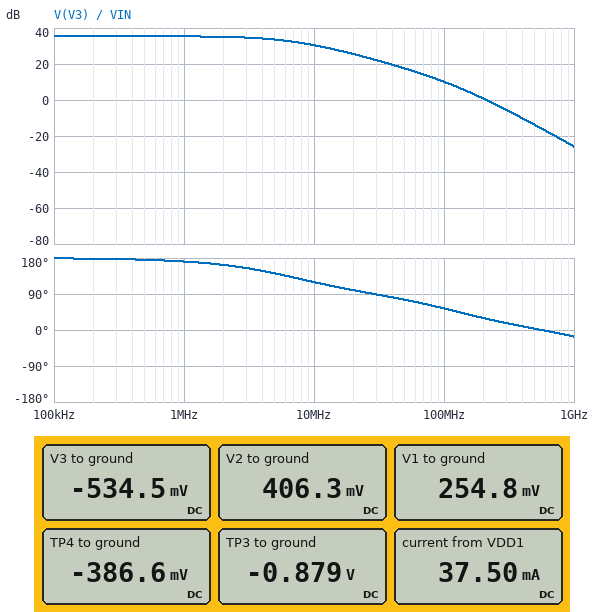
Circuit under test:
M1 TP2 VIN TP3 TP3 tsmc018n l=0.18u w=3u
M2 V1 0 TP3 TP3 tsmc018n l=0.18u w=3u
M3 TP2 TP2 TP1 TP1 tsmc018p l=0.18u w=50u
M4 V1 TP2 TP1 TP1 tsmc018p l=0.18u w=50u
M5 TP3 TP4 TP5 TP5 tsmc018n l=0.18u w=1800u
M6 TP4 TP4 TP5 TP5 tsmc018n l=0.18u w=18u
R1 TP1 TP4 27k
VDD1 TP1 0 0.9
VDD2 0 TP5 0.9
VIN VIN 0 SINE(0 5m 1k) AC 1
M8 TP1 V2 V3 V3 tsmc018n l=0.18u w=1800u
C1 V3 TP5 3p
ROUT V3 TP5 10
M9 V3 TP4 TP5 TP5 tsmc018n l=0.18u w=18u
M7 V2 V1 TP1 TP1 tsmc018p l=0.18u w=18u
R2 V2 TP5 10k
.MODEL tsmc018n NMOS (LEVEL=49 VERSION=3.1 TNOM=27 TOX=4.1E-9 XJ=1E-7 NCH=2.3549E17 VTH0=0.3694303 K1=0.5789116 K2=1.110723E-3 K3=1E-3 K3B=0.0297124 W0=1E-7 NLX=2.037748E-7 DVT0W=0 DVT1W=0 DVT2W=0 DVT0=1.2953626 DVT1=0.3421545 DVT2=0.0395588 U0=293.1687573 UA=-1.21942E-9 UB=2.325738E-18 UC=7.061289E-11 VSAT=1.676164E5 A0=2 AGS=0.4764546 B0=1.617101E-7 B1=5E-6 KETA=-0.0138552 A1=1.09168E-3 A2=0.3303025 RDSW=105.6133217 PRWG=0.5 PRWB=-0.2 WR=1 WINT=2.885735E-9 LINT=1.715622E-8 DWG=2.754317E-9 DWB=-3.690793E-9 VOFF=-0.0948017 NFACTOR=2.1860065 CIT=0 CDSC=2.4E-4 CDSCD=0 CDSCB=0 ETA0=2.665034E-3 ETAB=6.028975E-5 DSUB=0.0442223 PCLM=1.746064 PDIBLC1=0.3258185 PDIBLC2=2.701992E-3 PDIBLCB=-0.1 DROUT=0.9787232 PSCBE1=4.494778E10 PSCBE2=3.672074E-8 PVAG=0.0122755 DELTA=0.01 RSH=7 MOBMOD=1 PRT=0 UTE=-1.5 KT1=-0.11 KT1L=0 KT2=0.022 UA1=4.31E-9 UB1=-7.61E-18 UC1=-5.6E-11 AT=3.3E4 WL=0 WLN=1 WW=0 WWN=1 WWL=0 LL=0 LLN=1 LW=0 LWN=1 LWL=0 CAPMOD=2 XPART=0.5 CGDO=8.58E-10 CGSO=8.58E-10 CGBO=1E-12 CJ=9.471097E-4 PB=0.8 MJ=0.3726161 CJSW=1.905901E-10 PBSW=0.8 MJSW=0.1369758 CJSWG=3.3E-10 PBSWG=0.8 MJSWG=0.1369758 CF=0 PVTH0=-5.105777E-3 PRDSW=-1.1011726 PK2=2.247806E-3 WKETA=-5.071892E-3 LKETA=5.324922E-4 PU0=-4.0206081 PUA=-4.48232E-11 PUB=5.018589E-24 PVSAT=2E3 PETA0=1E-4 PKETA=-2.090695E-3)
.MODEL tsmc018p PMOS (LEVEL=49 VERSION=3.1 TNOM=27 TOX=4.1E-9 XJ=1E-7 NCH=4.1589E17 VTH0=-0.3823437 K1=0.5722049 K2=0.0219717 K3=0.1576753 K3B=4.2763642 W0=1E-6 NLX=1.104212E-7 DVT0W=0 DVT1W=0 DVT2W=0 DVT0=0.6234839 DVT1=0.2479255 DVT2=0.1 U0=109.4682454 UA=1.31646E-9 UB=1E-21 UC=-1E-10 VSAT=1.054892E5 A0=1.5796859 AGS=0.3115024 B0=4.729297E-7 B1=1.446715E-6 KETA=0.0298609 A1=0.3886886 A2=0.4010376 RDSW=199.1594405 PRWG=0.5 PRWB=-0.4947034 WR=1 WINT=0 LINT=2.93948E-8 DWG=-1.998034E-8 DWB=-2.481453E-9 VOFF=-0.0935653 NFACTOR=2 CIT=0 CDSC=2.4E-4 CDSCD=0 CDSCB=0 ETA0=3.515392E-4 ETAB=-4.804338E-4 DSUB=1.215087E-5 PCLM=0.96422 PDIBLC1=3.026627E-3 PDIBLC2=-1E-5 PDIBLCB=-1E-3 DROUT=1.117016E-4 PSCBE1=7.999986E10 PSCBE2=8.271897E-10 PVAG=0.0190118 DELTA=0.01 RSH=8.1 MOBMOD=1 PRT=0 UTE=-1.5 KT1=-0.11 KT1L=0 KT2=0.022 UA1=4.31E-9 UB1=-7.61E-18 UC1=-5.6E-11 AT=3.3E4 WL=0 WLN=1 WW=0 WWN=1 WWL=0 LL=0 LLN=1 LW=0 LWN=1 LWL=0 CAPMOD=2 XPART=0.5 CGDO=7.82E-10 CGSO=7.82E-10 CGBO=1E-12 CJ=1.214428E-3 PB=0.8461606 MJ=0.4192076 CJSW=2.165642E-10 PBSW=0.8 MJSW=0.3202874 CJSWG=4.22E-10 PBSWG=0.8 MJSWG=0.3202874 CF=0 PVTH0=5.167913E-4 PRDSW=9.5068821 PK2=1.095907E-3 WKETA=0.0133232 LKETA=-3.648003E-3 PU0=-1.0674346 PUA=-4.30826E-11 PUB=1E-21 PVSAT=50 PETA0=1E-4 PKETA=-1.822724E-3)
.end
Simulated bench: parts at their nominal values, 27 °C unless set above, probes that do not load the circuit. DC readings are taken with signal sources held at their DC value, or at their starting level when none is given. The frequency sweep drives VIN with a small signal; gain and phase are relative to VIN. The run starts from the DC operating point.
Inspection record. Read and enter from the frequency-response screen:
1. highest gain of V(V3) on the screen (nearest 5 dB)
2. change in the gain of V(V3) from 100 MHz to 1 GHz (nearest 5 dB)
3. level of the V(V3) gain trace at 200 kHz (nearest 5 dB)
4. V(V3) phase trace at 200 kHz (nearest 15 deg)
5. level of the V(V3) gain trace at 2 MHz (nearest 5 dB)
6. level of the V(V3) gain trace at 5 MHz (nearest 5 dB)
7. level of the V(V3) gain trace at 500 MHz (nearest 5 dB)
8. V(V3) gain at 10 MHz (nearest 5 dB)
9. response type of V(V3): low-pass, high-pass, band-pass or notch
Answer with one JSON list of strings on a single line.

["35 dB", "-35 dB", "35 dB", "180 deg", "35 dB", "35 dB", "-15 dB", "30 dB", "low-pass"]
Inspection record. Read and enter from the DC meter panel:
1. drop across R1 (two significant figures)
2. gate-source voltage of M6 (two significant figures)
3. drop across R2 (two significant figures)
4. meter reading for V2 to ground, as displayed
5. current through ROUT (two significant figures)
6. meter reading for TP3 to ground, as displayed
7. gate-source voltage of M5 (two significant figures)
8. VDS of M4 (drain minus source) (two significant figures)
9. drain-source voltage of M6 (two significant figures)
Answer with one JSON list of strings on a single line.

["1.3 V", "510 mV", "1.3 V", "406.3 mV", "37 mA", "-0.879 V", "510 mV", "-650 mV", "510 mV"]
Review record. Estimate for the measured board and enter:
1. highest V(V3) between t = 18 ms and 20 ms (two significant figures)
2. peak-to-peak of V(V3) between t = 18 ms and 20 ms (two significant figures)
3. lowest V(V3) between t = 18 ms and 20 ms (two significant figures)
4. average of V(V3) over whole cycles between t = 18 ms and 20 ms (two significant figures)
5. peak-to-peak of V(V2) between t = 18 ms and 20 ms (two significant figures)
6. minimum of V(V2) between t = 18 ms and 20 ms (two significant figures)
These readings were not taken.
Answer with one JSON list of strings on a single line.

["-370 mV", "440 mV", "-800 mV", "-560 mV", "960 mV", "-190 mV"]
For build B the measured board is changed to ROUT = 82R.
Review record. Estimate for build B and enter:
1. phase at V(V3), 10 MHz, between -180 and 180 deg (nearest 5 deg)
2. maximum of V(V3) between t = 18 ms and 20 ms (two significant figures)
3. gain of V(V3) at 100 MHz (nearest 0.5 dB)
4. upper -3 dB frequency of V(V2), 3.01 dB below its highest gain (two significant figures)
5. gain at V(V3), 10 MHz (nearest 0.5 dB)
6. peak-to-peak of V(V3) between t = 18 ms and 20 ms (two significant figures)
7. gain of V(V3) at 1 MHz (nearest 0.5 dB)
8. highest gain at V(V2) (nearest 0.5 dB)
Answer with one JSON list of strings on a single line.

["130 deg", "99 mV", "18.0 dB", "9.4 MHz", "37.0 dB", "780 mV", "40.5 dB", "42.0 dB"]
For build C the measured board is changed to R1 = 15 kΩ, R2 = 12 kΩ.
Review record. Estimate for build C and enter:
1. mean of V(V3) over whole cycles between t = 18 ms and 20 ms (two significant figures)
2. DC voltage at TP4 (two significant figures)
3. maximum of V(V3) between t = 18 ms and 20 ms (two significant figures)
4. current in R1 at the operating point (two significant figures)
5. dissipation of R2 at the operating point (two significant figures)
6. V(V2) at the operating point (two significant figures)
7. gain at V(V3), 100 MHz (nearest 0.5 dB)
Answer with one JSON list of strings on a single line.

["-500 mV", "-360 mV", "-350 mV", "84 µA", "190 µW", "600 mV", "9.5 dB"]
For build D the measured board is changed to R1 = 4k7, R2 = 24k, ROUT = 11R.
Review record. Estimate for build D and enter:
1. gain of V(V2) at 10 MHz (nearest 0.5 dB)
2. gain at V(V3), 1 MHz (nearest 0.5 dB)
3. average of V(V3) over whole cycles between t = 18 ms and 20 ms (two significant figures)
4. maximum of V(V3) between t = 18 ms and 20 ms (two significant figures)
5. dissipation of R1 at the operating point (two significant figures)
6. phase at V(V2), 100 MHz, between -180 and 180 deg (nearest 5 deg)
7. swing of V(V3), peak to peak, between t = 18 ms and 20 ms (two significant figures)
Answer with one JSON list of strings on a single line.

["18.0 dB", "12.0 dB", "-330 mV", "-300 mV", "300 µW", "75 deg", "120 mV"]
